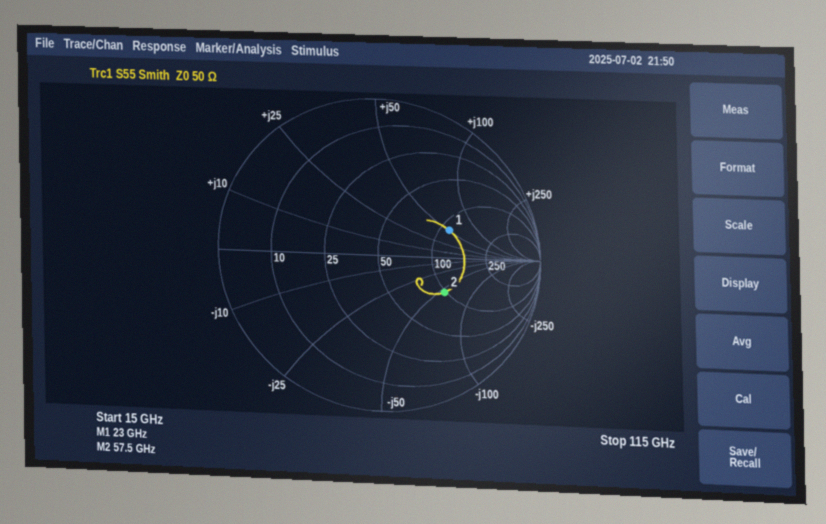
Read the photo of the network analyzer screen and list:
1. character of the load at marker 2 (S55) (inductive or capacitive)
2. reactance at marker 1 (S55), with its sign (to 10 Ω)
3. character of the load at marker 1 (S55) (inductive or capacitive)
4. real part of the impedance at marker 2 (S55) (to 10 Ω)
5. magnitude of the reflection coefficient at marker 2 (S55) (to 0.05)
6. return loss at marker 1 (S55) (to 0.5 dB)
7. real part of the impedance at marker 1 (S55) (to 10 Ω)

capacitive
+50 Ω
inductive
100 Ω
0.45
6.5 dB
110 Ω
